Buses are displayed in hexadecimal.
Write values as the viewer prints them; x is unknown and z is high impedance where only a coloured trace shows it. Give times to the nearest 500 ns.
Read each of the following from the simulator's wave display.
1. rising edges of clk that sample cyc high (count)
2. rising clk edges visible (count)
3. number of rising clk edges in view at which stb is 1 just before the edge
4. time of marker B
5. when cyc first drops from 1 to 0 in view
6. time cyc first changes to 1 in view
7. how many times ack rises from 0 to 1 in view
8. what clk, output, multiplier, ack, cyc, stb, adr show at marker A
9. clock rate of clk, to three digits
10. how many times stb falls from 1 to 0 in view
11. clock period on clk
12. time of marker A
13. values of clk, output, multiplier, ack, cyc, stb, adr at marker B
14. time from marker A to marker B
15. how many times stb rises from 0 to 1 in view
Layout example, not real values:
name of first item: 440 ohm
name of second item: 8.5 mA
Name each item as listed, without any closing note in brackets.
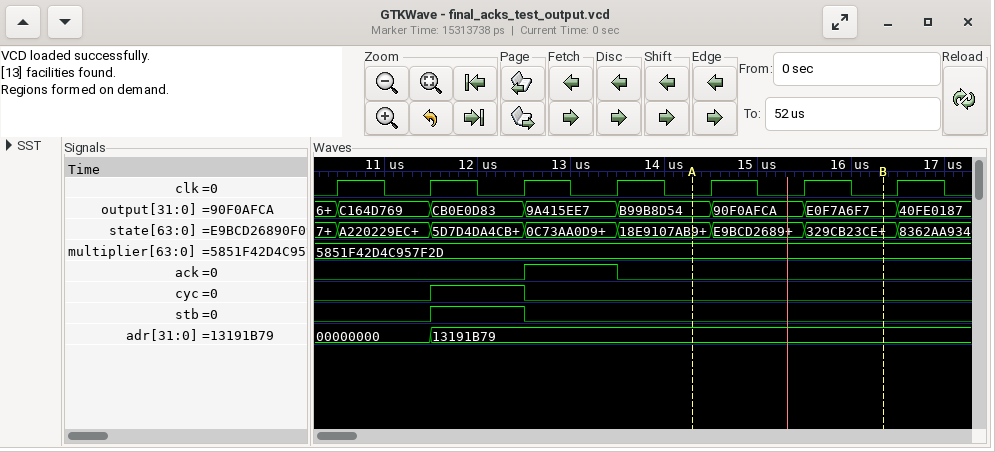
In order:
rising edges of clk that sample cyc high: 1
rising clk edges visible: 7
number of rising clk edges in view at which stb is 1 just before the edge: 1
time of marker B: 16500 ns
when cyc first drops from 1 to 0 in view: 12500 ns
time cyc first changes to 1 in view: 11500 ns
how many times ack rises from 0 to 1 in view: 1
what clk, output, multiplier, ack, cyc, stb, adr show at marker A: clk=0, output=B99B8D54, multiplier=5851F42D4C957F2D, ack=0, cyc=0, stb=0, adr=13191B79
clock rate of clk, to three digits: 1.00 MHz
how many times stb falls from 1 to 0 in view: 1
clock period on clk: 1000 ns
time of marker A: 14500 ns
values of clk, output, multiplier, ack, cyc, stb, adr at marker B: clk=0, output=E0F7A6F7, multiplier=5851F42D4C957F2D, ack=0, cyc=0, stb=0, adr=13191B79
time from marker A to marker B: 2000 ns
how many times stb rises from 0 to 1 in view: 1
